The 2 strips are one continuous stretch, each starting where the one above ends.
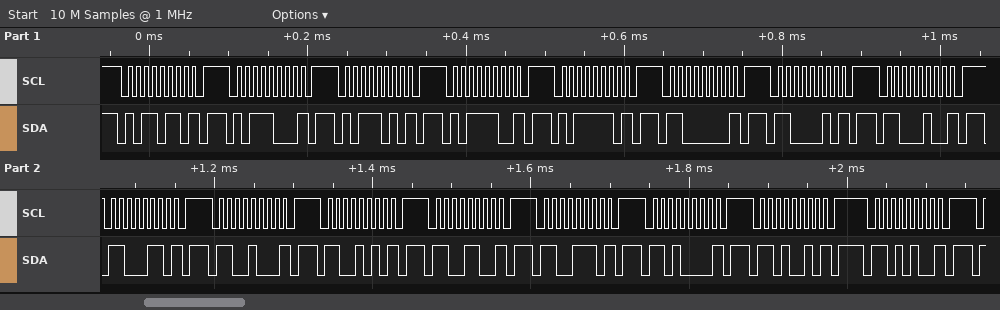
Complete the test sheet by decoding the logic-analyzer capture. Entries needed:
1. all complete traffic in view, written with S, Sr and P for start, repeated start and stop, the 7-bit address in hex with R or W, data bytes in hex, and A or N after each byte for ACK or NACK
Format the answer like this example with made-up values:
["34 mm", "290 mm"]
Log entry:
["S 5BW N P S 5CW N P S 5DW N P S 5EW N P S 5FW N P S 60W N P S 61W N P S 62W N P S 63W N P S 64W N P S 65W N P S 66W N P S 67W N P S 68W N P S 69W N P S 6AW N P"]
